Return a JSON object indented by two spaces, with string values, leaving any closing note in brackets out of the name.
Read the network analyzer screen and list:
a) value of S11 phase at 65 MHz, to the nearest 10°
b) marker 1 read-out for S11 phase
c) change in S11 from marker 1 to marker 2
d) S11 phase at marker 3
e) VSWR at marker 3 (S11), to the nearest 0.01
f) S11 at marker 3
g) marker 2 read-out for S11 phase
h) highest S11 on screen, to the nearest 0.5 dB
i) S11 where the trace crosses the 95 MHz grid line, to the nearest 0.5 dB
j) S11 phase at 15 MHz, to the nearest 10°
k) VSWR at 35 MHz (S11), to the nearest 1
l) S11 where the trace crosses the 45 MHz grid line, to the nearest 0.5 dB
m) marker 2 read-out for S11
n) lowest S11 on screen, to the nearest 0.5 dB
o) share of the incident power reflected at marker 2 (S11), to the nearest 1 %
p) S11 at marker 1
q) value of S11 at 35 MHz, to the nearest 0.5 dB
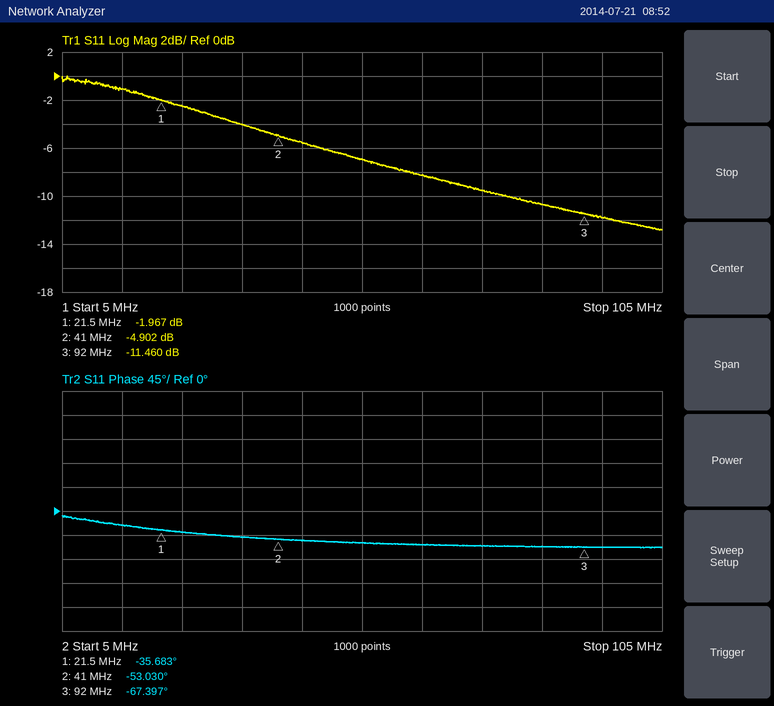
{
  "value of S11 phase at 65 MHz, to the nearest 10°": "-60°",
  "marker 1 read-out for S11 phase": "-35.683°",
  "change in S11 from marker 1 to marker 2": "-2.935 dB",
  "S11 phase at marker 3": "-67.397°",
  "VSWR at marker 3 (S11), to the nearest 0.01": "1.73",
  "S11 at marker 3": "-11.460 dB",
  "marker 2 read-out for S11 phase": "-53.030°",
  "highest S11 on screen, to the nearest 0.5 dB": "0.0 dB",
  "S11 where the trace crosses the 95 MHz grid line, to the nearest 0.5 dB": "-12.0 dB",
  "S11 phase at 15 MHz, to the nearest 10°": "-30°",
  "VSWR at 35 MHz (S11), to the nearest 1": "4",
  "S11 where the trace crosses the 45 MHz grid line, to the nearest 0.5 dB": "-5.5 dB",
  "marker 2 read-out for S11": "-4.902 dB",
  "lowest S11 on screen, to the nearest 0.5 dB": "-13.0 dB",
  "share of the incident power reflected at marker 2 (S11), to the nearest 1 %": "32 %",
  "S11 at marker 1": "-1.967 dB",
  "value of S11 at 35 MHz, to the nearest 0.5 dB": "-4.0 dB"
}
